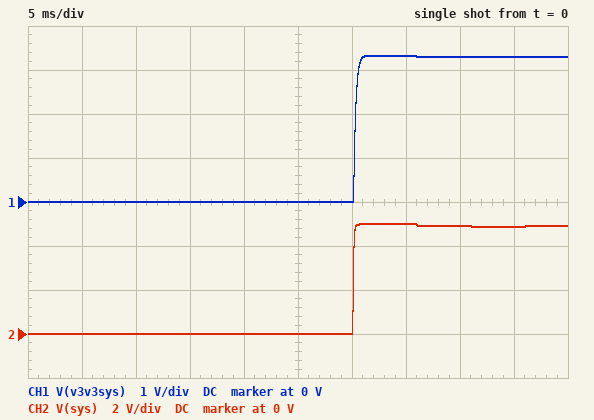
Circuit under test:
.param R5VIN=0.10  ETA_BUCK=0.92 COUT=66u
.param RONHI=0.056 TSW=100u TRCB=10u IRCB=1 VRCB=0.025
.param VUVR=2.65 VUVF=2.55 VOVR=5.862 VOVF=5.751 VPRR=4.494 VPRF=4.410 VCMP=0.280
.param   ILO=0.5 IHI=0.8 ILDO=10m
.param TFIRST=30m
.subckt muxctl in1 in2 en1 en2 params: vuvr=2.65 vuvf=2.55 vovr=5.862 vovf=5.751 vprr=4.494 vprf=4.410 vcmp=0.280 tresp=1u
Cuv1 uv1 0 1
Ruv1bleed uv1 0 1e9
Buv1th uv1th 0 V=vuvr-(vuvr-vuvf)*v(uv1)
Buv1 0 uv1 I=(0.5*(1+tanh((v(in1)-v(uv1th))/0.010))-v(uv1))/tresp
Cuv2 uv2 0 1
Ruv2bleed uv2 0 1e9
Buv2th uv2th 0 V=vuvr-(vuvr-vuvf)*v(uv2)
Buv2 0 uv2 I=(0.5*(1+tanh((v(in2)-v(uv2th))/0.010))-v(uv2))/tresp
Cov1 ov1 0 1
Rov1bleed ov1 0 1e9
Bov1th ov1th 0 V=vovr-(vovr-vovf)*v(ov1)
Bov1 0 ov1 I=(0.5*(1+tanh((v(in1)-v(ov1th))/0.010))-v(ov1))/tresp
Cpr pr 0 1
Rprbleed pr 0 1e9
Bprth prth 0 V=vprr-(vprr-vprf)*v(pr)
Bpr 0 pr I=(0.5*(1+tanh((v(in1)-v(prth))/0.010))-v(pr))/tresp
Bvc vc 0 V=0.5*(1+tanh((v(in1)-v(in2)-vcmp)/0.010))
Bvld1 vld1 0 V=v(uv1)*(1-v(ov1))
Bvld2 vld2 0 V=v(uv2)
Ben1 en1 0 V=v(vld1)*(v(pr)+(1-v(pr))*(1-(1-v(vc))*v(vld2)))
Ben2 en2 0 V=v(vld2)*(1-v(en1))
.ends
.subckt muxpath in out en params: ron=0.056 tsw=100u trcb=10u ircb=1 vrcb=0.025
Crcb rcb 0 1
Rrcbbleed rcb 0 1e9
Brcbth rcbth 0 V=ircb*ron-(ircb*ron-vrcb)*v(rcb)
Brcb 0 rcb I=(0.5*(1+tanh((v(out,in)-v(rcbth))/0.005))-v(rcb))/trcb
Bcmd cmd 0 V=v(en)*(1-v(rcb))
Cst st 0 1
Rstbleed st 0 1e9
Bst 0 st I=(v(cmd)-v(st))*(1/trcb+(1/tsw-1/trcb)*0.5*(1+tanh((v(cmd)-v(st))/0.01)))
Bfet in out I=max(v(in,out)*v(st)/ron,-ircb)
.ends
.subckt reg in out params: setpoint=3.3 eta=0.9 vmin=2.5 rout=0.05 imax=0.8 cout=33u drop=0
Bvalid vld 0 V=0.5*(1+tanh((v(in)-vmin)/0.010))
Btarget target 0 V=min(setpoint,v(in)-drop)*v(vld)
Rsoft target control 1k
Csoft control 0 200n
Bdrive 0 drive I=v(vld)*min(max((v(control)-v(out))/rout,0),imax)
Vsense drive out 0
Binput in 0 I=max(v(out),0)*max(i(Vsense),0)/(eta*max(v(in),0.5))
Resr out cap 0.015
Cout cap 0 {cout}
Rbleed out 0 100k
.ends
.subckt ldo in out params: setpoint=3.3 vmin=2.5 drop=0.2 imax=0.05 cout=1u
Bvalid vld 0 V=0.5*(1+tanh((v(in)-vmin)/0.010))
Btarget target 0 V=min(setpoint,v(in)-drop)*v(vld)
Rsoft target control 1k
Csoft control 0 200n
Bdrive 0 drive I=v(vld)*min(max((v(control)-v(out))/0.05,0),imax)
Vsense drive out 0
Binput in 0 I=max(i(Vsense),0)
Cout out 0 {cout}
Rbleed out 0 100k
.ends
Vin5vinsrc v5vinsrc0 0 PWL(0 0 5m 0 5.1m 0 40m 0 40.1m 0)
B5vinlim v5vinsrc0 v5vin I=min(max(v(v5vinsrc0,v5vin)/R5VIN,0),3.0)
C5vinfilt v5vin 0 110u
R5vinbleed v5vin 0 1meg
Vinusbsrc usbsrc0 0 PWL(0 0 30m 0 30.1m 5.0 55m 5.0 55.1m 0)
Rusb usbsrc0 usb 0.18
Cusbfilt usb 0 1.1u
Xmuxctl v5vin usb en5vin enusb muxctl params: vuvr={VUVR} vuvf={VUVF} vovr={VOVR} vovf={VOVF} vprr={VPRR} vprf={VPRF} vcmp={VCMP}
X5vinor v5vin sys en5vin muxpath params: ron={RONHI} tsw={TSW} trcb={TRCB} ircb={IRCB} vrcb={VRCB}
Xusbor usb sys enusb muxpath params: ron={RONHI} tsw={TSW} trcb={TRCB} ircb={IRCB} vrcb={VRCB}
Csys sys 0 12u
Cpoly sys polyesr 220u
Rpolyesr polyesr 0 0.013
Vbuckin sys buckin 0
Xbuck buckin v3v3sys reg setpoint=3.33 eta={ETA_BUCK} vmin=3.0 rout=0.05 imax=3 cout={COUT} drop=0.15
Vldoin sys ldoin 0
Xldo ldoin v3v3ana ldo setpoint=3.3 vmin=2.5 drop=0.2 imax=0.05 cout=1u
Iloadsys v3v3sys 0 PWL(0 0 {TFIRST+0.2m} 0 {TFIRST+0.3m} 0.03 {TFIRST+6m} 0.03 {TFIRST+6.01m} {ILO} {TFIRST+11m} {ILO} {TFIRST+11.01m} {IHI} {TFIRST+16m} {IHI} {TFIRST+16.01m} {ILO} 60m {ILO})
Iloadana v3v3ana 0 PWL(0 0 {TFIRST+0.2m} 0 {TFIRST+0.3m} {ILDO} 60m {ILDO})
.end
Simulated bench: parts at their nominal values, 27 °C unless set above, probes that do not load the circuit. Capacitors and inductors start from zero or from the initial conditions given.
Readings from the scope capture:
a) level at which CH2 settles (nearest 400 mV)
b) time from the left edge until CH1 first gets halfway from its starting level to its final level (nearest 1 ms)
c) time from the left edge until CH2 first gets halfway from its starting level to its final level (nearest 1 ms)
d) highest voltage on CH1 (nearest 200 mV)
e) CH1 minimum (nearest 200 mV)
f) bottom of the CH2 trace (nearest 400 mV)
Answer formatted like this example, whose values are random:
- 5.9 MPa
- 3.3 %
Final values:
- 4.8 V
- 30 ms
- 30 ms
- 3.4 V
- 0 V
- 0 V
